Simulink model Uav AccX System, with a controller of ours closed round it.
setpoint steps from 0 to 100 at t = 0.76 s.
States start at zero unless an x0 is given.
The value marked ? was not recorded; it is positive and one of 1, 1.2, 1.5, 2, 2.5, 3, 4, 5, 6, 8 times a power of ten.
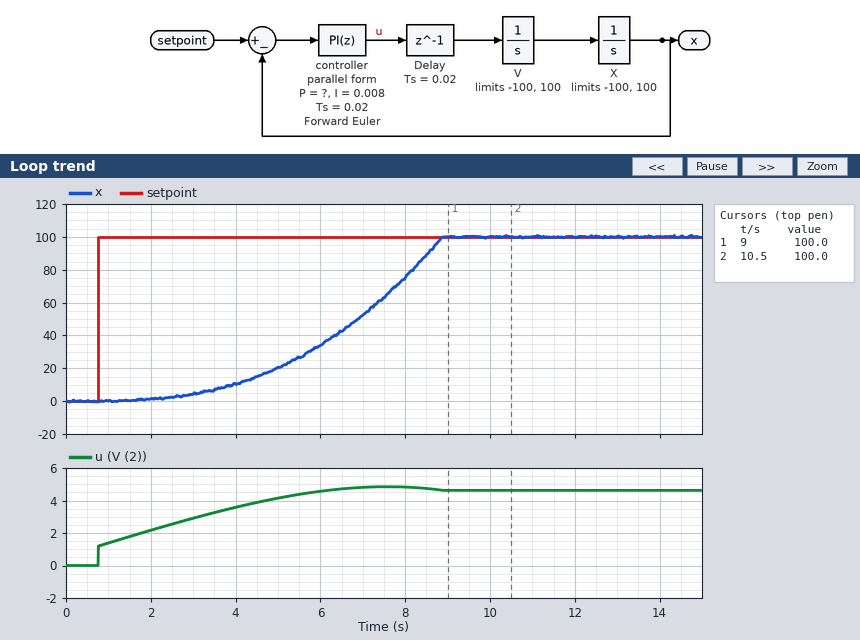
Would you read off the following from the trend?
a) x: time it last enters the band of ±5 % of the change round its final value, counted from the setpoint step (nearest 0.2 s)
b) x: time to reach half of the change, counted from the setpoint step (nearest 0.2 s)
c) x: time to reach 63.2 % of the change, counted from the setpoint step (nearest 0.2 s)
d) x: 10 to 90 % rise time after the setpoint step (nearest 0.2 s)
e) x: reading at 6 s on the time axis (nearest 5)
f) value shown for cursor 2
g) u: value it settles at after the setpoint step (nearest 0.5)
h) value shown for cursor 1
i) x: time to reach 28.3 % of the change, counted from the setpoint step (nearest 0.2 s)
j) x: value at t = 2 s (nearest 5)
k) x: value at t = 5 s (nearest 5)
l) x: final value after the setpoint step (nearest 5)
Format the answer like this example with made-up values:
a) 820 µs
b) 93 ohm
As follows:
a) 8.0 s
b) 6.2 s
c) 6.8 s
d) 4.6 s
e) 35
f) 100.0
g) 4.5
h) 100.0
i) 4.8 s
j) 0
k) 20
l) 100
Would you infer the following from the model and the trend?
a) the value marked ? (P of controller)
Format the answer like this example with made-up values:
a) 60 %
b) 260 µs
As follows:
a) 0.012
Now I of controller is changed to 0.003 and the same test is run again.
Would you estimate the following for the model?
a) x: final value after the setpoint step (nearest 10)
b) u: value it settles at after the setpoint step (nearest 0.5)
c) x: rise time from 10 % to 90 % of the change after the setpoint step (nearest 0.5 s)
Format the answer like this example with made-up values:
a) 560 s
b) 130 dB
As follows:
a) 100
b) 2.0
c) 6.0 s
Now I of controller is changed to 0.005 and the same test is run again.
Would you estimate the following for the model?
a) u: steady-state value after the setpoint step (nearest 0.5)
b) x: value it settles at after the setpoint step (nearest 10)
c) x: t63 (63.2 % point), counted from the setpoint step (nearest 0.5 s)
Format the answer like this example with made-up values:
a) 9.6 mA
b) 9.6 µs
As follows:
a) 3.0
b) 100
c) 7.5 s
